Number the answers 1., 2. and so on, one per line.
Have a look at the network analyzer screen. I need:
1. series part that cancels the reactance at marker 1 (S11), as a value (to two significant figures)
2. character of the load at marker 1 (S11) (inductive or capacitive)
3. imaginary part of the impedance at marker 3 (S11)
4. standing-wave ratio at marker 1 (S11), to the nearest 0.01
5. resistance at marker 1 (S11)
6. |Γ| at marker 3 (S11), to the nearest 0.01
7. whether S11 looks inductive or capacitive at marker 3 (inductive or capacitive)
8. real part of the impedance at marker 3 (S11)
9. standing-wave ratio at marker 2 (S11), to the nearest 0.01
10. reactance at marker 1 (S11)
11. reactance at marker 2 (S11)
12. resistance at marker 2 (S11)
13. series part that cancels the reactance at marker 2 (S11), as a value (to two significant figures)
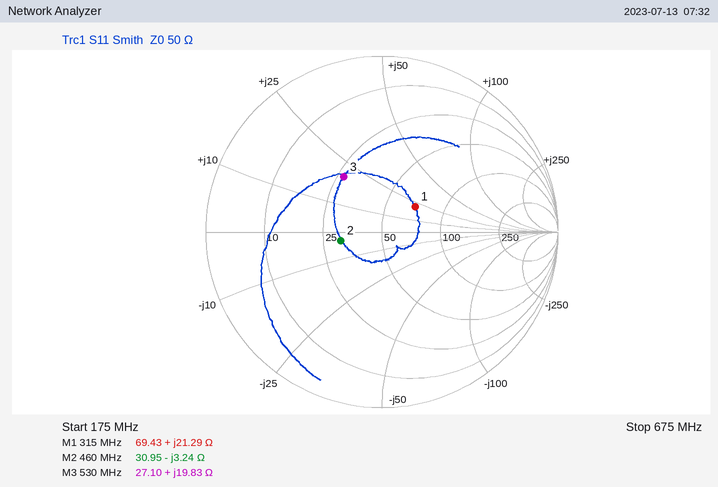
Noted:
1. 24 pF
2. inductive
3. +19.83 Ω
4. 1.62
5. 69.43 Ω
6. 0.38
7. inductive
8. 27.10 Ω
9. 1.63
10. +21.29 Ω
11. -3.24 Ω
12. 30.95 Ω
13. 1.1 nH
